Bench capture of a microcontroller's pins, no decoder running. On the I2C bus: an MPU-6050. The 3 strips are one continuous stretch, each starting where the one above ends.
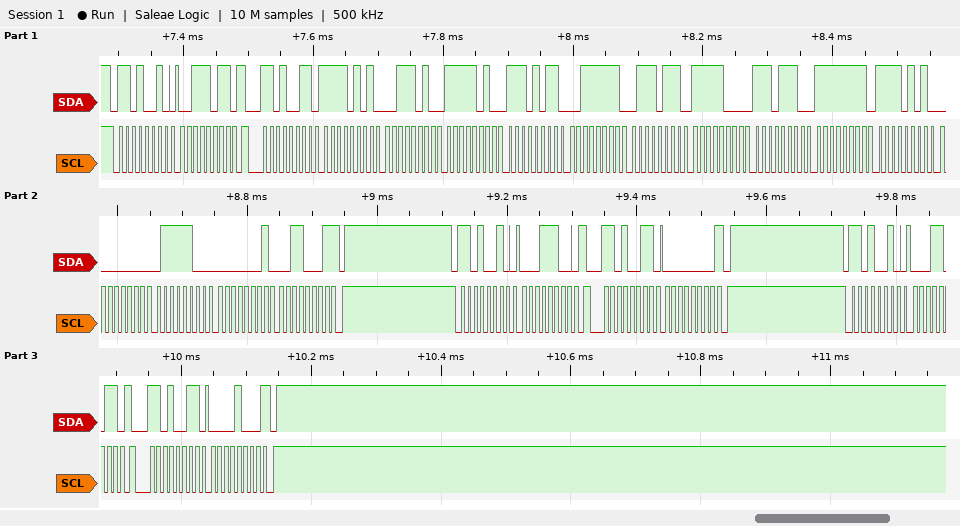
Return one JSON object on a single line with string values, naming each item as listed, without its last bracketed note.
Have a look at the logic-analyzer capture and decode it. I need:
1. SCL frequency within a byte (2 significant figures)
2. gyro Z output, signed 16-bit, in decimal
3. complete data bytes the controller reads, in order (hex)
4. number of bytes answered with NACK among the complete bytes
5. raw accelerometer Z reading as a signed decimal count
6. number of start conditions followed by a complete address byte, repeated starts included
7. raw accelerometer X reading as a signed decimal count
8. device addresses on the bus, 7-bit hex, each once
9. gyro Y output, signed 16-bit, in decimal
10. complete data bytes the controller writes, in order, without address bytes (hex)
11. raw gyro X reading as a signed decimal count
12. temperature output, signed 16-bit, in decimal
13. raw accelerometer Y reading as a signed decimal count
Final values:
{"SCL frequency within a byte": "100 kHz", "gyro Z output, signed 16-bit, in decimal": "305", "complete data bytes the controller reads, in order": "F5 3A FA EB 3F 77 F8 EE FF F5 00 7C 01 31 00 08", "number of bytes answered with NACK among the complete bytes": "3", "raw accelerometer Z reading as a signed decimal count": "16247", "number of start conditions followed by a complete address byte, repeated starts included": "6", "raw accelerometer X reading as a signed decimal count": "-2758", "device addresses on the bus, 7-bit hex, each once": "0x69", "gyro Y output, signed 16-bit, in decimal": "124", "complete data bytes the controller writes, in order, without address bytes": "3B 1C 1B", "raw gyro X reading as a signed decimal count": "-11", "temperature output, signed 16-bit, in decimal": "-1810", "raw accelerometer Y reading as a signed decimal count": "-1301"}
